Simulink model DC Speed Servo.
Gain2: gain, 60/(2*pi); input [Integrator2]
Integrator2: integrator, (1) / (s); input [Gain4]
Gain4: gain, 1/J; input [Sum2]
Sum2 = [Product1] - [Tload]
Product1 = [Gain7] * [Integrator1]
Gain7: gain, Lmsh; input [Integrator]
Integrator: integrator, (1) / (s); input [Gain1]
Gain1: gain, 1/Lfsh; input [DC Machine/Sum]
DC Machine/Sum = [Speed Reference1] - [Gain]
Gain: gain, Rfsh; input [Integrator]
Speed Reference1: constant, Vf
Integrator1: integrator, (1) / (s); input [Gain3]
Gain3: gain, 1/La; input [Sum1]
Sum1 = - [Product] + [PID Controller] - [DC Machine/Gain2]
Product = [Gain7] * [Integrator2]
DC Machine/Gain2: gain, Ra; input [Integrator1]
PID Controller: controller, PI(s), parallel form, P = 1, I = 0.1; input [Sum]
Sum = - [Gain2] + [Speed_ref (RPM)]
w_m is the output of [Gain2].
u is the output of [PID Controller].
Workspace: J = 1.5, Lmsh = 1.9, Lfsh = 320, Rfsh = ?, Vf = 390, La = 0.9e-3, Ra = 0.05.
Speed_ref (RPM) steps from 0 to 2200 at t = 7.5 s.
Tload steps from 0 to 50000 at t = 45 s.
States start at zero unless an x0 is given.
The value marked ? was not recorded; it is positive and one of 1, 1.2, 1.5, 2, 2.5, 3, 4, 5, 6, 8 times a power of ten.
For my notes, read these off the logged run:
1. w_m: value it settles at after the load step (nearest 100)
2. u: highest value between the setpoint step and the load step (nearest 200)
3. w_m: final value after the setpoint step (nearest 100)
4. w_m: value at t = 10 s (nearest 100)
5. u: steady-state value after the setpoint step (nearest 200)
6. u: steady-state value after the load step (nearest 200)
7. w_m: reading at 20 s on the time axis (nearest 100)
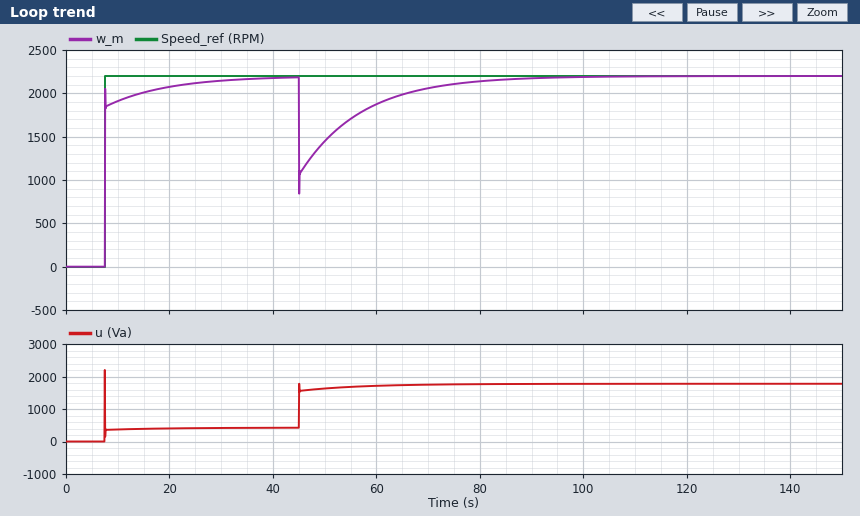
2200
2200
2200
1900
400
1800
2100
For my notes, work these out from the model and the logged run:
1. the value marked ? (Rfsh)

400
